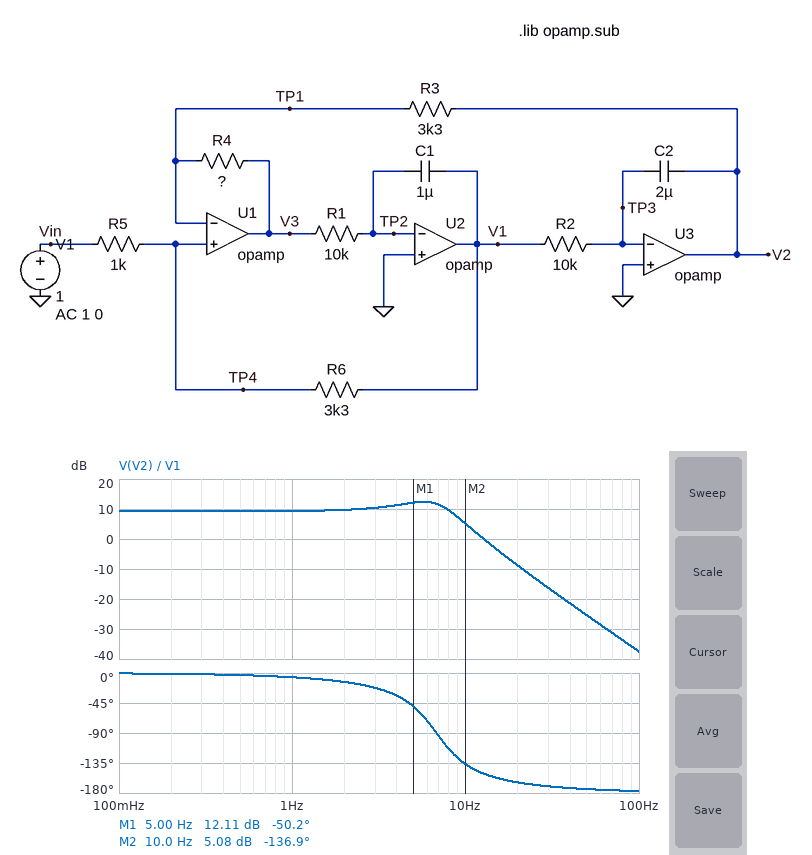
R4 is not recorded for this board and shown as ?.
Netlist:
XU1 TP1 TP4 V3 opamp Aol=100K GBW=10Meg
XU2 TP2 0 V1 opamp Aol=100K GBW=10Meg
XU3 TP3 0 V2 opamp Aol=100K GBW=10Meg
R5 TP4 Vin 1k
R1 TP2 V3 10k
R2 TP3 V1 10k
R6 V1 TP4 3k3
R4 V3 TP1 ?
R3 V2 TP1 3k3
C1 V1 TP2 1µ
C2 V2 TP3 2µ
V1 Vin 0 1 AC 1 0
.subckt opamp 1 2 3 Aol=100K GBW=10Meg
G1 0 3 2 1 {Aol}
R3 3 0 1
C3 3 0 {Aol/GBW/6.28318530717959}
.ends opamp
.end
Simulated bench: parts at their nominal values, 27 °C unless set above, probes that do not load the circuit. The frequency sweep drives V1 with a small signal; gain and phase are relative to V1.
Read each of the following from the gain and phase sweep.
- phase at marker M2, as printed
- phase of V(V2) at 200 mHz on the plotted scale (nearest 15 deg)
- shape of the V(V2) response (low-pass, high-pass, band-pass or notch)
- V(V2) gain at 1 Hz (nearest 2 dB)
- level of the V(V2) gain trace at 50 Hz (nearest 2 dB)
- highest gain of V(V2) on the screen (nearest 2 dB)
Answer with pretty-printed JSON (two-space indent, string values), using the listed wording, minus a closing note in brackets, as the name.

{
  "phase at marker M2, as printed": "-136.9 deg",
  "phase of V(V2) at 200 mHz on the plotted scale": "0 deg",
  "shape of the V(V2) response": "low-pass",
  "V(V2) gain at 1 Hz": "10 dB",
  "level of the V(V2) gain trace at 50 Hz": "-26 dB",
  "highest gain of V(V2) on the screen": "12 dB"
}
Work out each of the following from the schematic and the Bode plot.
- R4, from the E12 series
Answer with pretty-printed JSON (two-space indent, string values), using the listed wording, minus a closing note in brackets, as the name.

{
  "R4, from the E12 series": "1.2 kΩ"
}
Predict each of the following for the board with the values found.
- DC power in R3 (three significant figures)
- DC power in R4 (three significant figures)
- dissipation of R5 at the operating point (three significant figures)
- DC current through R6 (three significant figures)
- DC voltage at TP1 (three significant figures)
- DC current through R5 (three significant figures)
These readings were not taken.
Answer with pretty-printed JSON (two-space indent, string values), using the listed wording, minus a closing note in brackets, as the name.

{
  "DC power in R3": "1.35 mW",
  "DC power in R4": "491 µW",
  "dissipation of R5 at the operating point": "54.1 µW",
  "DC current through R6": "233 µA",
  "DC voltage at TP1": "767 mV",
  "DC current through R5": "233 µA"
}
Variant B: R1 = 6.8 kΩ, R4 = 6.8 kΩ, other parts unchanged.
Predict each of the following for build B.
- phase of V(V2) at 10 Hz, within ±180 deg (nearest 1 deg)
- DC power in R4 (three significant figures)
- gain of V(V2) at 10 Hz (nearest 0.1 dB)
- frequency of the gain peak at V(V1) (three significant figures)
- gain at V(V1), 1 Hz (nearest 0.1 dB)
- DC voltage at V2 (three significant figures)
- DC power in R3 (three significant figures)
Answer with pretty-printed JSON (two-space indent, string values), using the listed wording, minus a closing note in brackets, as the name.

{
  "phase of V(V2) at 10 Hz, within ±180 deg": "-30 deg",
  "DC power in R4": "86.6 µW",
  "gain of V(V2) at 10 Hz": "2.5 dB",
  "frequency of the gain peak at V(V1)": "19.6 Hz",
  "gain at V(V1), 1 Hz": "-16.9 dB",
  "DC voltage at V2": "1.14 V",
  "DC power in R3": "42.0 µW"
}
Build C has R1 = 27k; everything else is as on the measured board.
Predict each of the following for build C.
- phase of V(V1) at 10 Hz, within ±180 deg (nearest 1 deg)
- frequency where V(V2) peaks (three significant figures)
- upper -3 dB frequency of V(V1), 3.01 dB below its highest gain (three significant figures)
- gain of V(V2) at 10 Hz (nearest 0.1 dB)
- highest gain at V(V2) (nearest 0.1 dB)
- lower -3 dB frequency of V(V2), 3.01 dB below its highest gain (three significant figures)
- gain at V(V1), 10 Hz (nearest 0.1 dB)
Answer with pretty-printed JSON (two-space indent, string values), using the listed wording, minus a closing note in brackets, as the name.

{
  "phase of V(V1) at 10 Hz, within ±180 deg": "103 deg",
  "frequency where V(V2) peaks": "3.91 Hz",
  "upper -3 dB frequency of V(V1), 3.01 dB below its highest gain": "5.17 Hz",
  "gain of V(V2) at 10 Hz": "-4.8 dB",
  "highest gain at V(V2)": "16.3 dB",
  "lower -3 dB frequency of V(V2), 3.01 dB below its highest gain": "2.79 Hz",
  "gain at V(V1), 10 Hz": "-2.8 dB"
}
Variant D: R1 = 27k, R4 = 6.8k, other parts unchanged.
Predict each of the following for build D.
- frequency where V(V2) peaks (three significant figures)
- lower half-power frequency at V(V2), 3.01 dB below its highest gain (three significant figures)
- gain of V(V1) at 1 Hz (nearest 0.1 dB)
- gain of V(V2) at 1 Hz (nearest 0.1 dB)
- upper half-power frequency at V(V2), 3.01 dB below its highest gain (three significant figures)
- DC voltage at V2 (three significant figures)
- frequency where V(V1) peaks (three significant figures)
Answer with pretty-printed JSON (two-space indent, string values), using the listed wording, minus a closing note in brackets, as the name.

{
  "frequency where V(V2) peaks": "9.37 Hz",
  "lower half-power frequency at V(V2), 3.01 dB below its highest gain": "6.90 Hz",
  "gain of V(V1) at 1 Hz": "-16.8 dB",
  "gain of V(V2) at 1 Hz": "1.2 dB",
  "upper half-power frequency at V(V2), 3.01 dB below its highest gain": "11.3 Hz",
  "DC voltage at V2": "1.14 V",
  "frequency where V(V1) peaks": "9.83 Hz"
}
